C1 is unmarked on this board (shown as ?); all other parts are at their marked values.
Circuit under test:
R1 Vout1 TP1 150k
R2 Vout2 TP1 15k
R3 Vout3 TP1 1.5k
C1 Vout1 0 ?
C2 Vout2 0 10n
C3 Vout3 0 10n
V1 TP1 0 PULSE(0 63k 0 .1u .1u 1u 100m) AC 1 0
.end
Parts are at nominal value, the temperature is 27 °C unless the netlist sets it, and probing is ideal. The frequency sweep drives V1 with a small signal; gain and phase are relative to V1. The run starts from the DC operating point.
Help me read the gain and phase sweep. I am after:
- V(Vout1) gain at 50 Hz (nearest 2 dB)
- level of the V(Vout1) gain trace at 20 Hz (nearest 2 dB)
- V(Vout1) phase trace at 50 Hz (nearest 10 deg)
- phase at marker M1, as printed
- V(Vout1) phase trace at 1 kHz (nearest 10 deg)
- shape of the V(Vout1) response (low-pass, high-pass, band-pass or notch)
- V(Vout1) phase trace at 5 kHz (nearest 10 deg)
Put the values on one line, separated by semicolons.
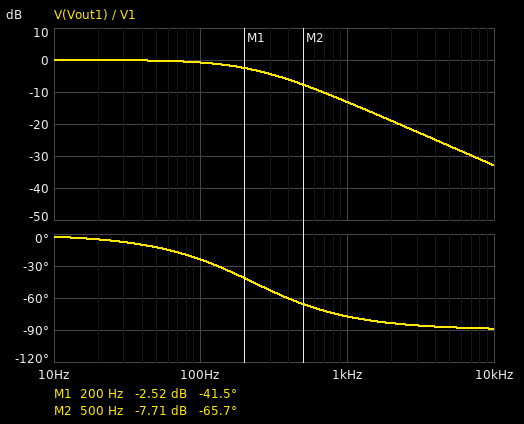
0 dB; 0 dB; -10 deg; -41.5 deg; -80 deg; low-pass; -90 deg
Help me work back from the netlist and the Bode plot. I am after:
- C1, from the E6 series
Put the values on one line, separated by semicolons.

4.7 nF
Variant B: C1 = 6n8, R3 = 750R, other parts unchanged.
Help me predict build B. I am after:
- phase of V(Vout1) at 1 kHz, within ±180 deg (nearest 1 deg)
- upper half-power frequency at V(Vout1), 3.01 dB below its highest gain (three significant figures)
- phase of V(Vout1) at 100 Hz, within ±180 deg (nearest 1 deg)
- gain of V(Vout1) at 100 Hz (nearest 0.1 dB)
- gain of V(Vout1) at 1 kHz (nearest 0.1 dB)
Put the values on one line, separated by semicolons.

-81 deg; 156 Hz; -33 deg; -1.5 dB; -16.2 dB
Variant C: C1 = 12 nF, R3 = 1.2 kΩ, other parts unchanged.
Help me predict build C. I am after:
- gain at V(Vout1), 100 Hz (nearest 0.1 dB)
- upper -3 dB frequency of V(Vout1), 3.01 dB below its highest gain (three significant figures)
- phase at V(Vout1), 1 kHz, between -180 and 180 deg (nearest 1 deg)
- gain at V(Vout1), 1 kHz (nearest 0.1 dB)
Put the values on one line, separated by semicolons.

-3.6 dB; 88.4 Hz; -85 deg; -21.1 dB
